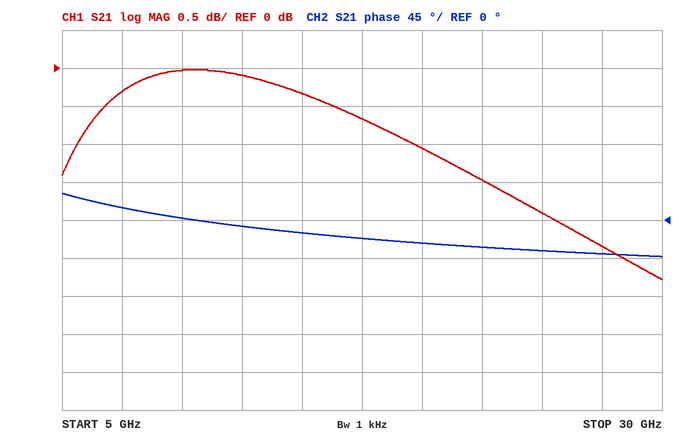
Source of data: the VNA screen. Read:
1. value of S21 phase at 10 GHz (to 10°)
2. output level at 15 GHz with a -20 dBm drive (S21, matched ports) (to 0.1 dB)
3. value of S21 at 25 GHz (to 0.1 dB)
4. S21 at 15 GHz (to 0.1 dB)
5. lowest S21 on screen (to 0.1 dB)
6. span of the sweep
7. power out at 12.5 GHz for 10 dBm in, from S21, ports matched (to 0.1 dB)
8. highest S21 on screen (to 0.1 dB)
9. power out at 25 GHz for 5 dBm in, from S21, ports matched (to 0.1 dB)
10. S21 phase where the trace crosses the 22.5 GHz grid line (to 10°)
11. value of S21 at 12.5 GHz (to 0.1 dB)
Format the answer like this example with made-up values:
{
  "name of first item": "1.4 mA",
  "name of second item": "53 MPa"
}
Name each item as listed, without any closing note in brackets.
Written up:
{
  "value of S21 phase at 10 GHz": "0°",
  "output level at 15 GHz with a -20 dBm drive (S21, matched ports)": "-20.3 dBm",
  "value of S21 at 25 GHz": "-1.9 dB",
  "S21 at 15 GHz": "-0.3 dB",
  "lowest S21 on screen": "-2.8 dB",
  "span of the sweep": "25 GHz",
  "power out at 12.5 GHz for 10 dBm in, from S21, ports matched": "9.9 dBm",
  "highest S21 on screen": "0.0 dB",
  "power out at 25 GHz for 5 dBm in, from S21, ports matched": "3.1 dBm",
  "S21 phase where the trace crosses the 22.5 GHz grid line": "-30°",
  "value of S21 at 12.5 GHz": "-0.1 dB"
}
